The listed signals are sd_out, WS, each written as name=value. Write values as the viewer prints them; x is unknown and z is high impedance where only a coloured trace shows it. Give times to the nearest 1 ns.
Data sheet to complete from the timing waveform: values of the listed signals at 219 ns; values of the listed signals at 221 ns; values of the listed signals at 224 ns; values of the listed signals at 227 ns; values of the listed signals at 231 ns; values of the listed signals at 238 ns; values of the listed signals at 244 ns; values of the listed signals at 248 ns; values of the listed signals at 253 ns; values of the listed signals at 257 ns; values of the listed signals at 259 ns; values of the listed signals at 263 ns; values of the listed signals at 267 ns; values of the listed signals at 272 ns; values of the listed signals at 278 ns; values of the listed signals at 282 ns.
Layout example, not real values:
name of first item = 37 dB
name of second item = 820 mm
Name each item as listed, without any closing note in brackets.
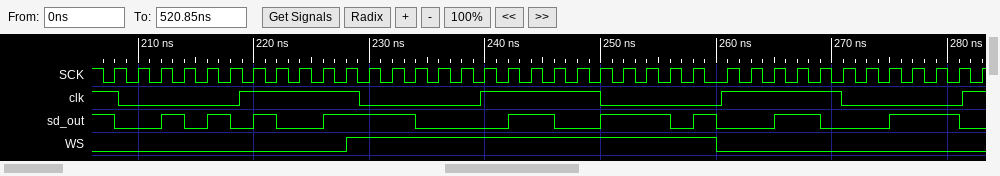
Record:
values of the listed signals at 219 ns = sd_out=0, WS=0
values of the listed signals at 221 ns = sd_out=1, WS=0
values of the listed signals at 224 ns = sd_out=0, WS=0
values of the listed signals at 227 ns = sd_out=1, WS=0
values of the listed signals at 231 ns = sd_out=1, WS=1
values of the listed signals at 238 ns = sd_out=0, WS=1
values of the listed signals at 244 ns = sd_out=1, WS=1
values of the listed signals at 248 ns = sd_out=0, WS=1
values of the listed signals at 253 ns = sd_out=1, WS=1
values of the listed signals at 257 ns = sd_out=0, WS=1
values of the listed signals at 259 ns = sd_out=1, WS=1
values of the listed signals at 263 ns = sd_out=0, WS=0
values of the listed signals at 267 ns = sd_out=1, WS=0
values of the listed signals at 272 ns = sd_out=0, WS=0
values of the listed signals at 278 ns = sd_out=1, WS=0
values of the listed signals at 282 ns = sd_out=0, WS=0
